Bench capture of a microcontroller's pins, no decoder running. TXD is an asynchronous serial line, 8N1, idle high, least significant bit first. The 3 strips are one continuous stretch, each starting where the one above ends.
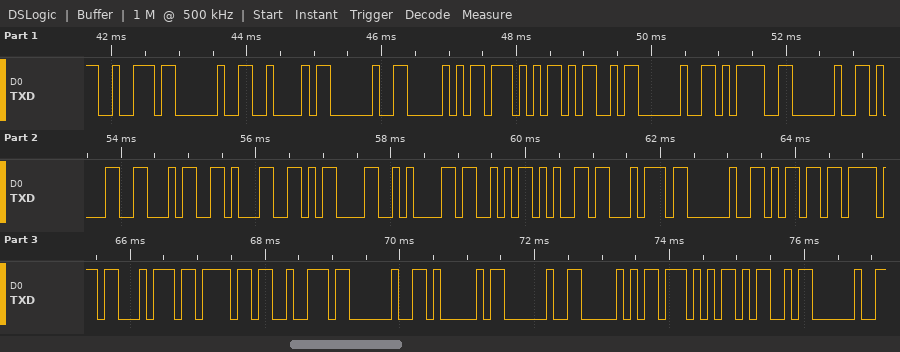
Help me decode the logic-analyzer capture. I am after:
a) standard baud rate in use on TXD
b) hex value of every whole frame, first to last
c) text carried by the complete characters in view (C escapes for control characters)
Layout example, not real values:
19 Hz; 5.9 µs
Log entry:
9600 baud; 72 20 42 20 50 57 4D 20 3D 20 31 34 31 0D 0A 53 65 74 20 6D 6F 74 6F 72 20 41 20 50 57 4D 20; "r B PWM = 141\r\nSet motor A PWM "
